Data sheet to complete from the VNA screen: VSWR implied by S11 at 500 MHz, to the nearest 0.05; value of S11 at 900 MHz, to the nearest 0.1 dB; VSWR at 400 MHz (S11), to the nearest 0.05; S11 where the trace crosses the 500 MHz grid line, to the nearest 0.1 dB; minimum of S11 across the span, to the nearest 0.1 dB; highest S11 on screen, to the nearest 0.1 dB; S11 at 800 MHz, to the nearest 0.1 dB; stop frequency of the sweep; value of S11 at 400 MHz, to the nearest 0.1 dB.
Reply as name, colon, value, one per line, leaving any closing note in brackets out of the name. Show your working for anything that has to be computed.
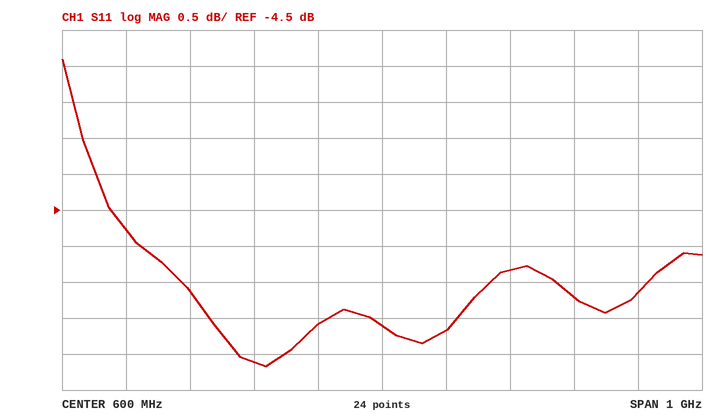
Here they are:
VSWR implied by S11 at 500 MHz, to the nearest 0.05: |Γ| = 10^(-6.1/20) = 0.4955; VSWR = (1 + 0.4955)/(1 − 0.4955) ≈ 2.96, so 2.95 to the nearest 0.05
value of S11 at 900 MHz, to the nearest 0.1 dB: -5.7 dB
VSWR at 400 MHz (S11), to the nearest 0.05: |Γ| = 10^(-6.6/20) = 0.4677; VSWR = (1 + 0.4677)/(1 − 0.4677) ≈ 2.76, so 2.75 to the nearest 0.05
S11 where the trace crosses the 500 MHz grid line, to the nearest 0.1 dB: -6.1 dB
minimum of S11 across the span, to the nearest 0.1 dB: -6.7 dB
highest S11 on screen, to the nearest 0.1 dB: -2.4 dB
S11 at 800 MHz, to the nearest 0.1 dB: -5.3 dB
stop frequency of the sweep: 1.1 GHz
value of S11 at 400 MHz, to the nearest 0.1 dB: -6.6 dB
